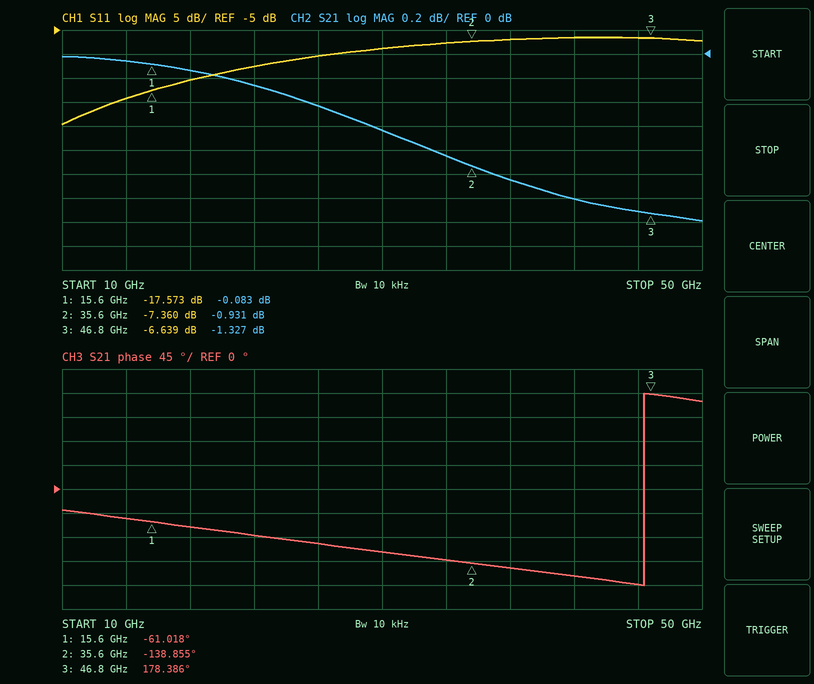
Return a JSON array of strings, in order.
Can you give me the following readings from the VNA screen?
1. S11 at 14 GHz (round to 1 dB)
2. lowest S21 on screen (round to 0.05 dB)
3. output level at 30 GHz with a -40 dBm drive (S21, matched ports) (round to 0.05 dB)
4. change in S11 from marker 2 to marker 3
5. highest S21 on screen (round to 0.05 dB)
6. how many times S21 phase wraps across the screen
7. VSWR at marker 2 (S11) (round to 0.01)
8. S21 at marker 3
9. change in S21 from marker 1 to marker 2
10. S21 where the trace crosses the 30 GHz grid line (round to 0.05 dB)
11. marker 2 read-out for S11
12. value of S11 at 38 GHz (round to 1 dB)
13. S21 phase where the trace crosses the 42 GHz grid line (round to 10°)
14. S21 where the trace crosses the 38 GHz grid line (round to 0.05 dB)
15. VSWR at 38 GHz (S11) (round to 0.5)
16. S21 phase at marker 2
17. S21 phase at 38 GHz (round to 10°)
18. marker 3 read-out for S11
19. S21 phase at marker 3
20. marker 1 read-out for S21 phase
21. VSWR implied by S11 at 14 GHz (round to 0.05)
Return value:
["-19 dB", "-1.40 dB", "-40.65 dBm", "0.721 dB", "0.00 dB", "1", "2.50", "-1.327 dB", "-0.848 dB", "-0.65 dB", "-7.360 dB", "-7 dB", "-160°", "-1.05 dB", "2.5", "-138.855°", "-150°", "-6.639 dB", "178.386°", "-61.018°", "1.25"]
